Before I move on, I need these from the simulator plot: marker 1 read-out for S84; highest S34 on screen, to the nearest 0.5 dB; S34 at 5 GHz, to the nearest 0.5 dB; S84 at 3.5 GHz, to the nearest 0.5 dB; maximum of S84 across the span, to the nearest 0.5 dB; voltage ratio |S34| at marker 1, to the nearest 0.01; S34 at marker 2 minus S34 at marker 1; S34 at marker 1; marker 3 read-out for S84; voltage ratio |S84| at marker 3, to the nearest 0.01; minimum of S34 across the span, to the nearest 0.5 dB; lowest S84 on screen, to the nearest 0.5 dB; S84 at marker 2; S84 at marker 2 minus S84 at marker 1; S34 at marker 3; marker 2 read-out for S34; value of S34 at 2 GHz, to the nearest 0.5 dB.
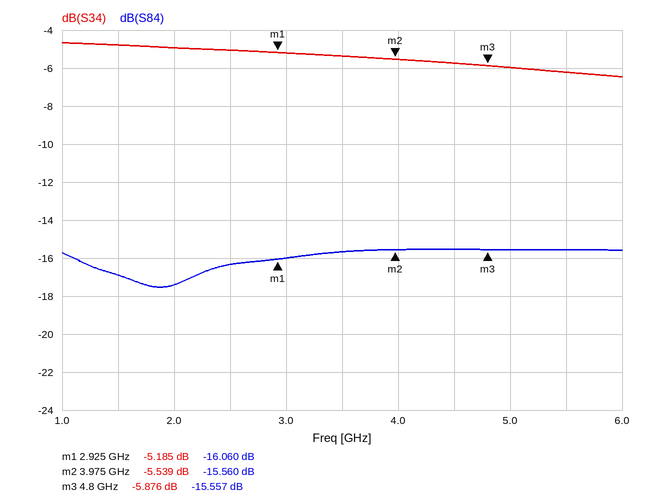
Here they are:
-16.060 dB
-4.5 dB
-6.0 dB
-15.5 dB
-15.5 dB
0.55
-0.354 dB
-5.185 dB
-15.557 dB
0.17
-6.5 dB
-17.5 dB
-15.560 dB
0.500 dB
-5.876 dB
-5.539 dB
-5.0 dB
